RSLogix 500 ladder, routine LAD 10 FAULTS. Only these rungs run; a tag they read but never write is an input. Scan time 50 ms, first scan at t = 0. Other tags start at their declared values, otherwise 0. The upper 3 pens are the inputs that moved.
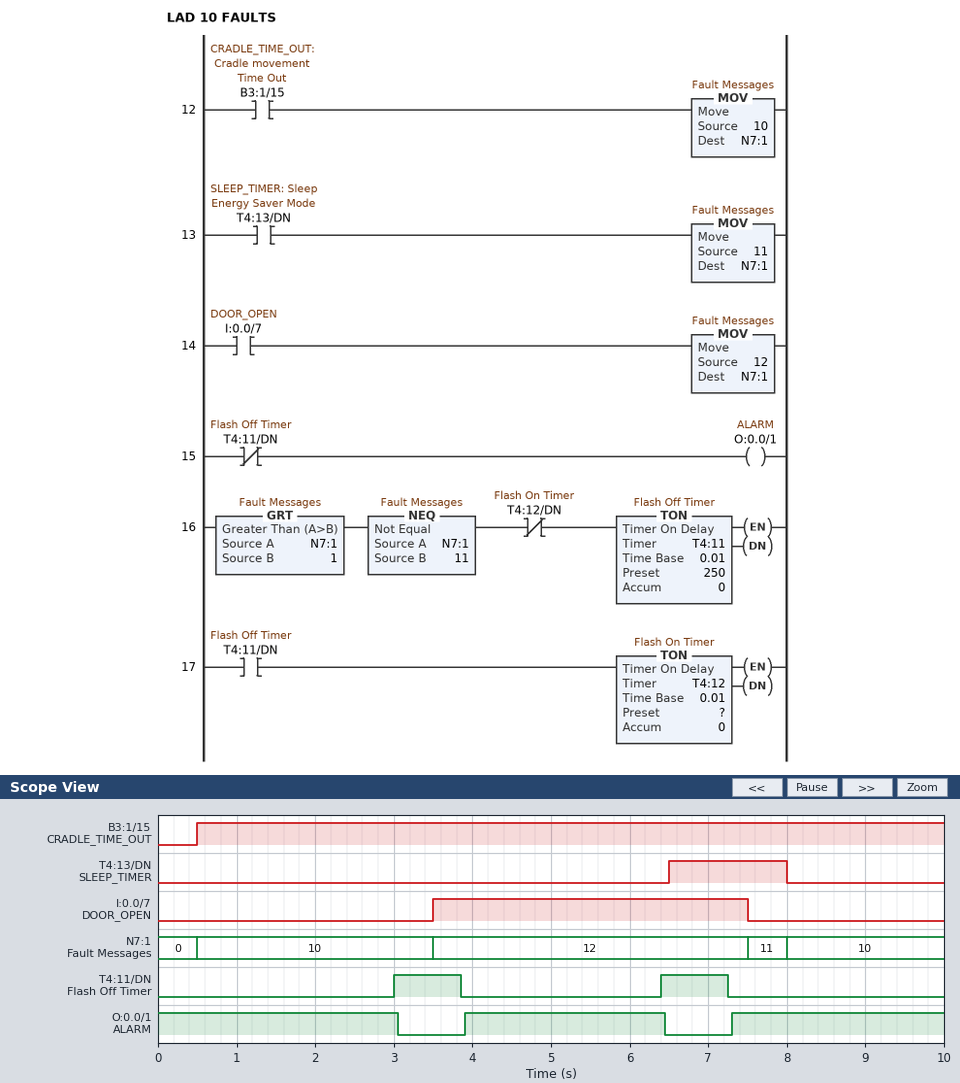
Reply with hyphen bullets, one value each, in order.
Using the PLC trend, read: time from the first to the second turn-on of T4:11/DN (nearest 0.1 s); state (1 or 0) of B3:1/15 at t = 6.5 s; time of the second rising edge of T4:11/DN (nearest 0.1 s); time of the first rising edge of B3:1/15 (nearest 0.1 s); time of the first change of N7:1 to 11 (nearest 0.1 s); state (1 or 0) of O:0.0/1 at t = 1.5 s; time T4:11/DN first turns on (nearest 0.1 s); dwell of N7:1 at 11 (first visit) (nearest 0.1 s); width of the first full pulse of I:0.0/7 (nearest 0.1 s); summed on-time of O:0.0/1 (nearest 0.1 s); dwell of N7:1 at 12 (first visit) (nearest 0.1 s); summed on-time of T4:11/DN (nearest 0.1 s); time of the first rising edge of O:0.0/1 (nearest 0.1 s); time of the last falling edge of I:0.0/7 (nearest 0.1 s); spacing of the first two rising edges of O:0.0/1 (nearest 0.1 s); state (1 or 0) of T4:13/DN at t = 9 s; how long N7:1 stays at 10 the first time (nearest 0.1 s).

- 3.4 s
- 1
- 6.4 s
- 0.5 s
- 7.5 s
- 1
- 3.0 s
- 0.5 s
- 4.0 s
- 8.3 s
- 4.0 s
- 1.7 s
- 3.9 s
- 7.5 s
- 3.4 s
- 0
- 3.0 s
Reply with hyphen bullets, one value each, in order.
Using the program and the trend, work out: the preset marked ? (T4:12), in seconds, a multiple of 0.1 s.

- 0.8 s
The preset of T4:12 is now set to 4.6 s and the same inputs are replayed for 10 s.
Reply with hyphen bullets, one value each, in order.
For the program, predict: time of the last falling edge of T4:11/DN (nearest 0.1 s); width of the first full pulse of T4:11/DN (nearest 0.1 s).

- 7.5 s
- 4.5 s
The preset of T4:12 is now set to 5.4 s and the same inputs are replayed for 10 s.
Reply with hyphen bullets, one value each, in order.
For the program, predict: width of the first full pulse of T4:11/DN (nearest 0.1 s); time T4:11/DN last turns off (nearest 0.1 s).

- 4.5 s
- 7.5 s
